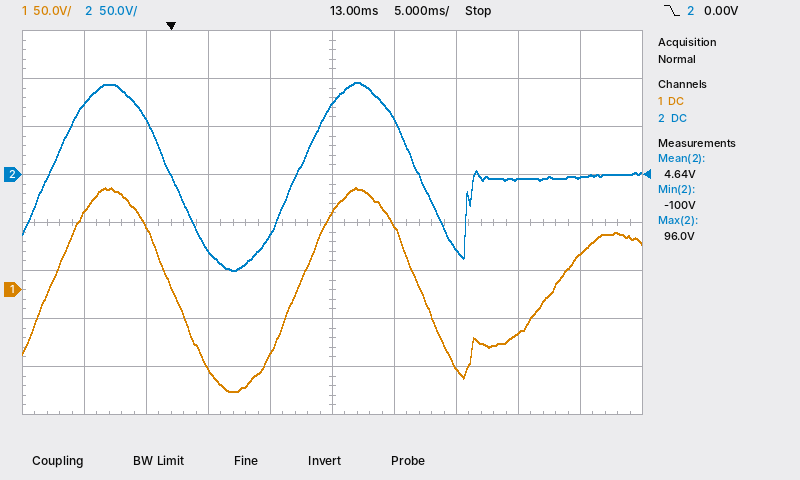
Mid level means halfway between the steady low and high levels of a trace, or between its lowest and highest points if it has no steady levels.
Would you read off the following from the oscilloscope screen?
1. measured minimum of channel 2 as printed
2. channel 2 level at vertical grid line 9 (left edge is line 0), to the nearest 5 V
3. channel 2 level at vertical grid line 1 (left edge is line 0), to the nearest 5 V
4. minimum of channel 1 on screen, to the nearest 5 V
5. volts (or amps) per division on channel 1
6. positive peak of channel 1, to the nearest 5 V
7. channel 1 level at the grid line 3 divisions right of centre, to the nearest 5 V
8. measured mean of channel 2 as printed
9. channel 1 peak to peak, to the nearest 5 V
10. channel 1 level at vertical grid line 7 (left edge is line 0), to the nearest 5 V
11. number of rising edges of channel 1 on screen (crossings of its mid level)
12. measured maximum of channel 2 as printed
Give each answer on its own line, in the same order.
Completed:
-100 V
-5 V
75 V
-105 V
50 V
105 V
-45 V
4.64 V
210 V
-80 V
3
96.0 V
